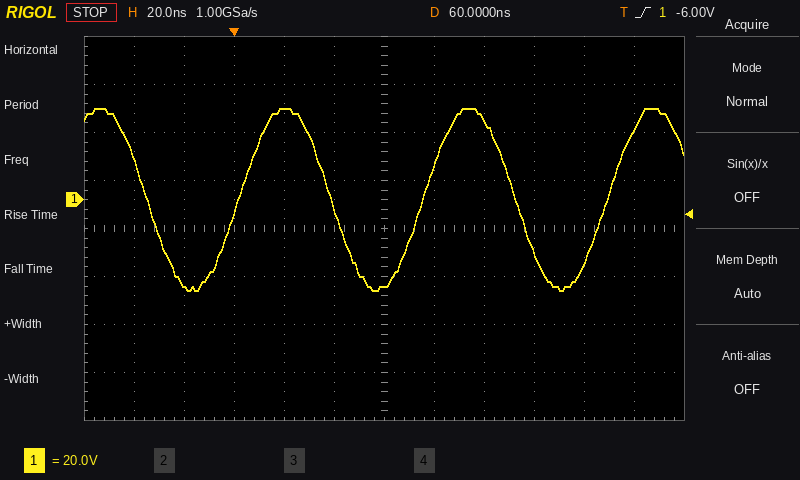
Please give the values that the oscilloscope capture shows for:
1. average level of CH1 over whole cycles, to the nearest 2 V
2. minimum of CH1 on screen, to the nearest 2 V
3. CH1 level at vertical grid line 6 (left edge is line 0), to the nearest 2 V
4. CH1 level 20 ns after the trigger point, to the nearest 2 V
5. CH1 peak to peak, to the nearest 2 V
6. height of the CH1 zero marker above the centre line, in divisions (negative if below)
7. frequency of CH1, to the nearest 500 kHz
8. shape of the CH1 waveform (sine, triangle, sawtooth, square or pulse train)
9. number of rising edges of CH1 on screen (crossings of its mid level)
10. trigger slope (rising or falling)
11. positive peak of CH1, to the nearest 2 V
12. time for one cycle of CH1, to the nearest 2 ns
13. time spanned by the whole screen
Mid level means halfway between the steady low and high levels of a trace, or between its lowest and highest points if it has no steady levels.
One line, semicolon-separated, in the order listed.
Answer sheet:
0 V; -38 V; -36 V; 38 V; 76 V; +0.6 div; 13.5 MHz; sine; 3; rising; 38 V; 74 ns; 240 ns
